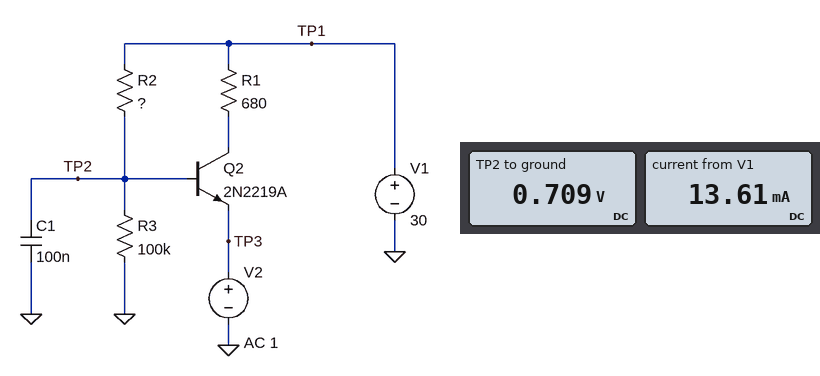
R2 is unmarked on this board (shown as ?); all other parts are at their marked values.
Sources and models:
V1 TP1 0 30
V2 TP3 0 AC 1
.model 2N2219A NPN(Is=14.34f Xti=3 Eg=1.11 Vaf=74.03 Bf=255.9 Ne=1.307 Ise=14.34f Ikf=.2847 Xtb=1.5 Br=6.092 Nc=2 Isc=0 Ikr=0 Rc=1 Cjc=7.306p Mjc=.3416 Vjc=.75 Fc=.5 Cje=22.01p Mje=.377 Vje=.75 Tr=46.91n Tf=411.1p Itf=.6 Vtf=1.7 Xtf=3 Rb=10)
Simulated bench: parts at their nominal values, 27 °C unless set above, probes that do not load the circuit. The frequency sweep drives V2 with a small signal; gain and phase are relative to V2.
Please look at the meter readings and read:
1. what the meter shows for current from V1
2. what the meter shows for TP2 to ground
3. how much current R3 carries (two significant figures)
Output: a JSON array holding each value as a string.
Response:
["13.61 mA", "0.709 V", "7.1 µA"]
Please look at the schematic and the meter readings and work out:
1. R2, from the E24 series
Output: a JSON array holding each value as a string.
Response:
["430 kΩ"]
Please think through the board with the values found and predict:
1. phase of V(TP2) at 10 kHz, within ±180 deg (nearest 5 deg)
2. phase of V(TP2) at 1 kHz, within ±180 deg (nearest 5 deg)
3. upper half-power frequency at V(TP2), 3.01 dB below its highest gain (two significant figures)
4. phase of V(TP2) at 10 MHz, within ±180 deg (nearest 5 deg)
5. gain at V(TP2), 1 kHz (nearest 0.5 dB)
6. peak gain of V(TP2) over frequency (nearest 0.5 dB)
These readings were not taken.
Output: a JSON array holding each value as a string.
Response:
["-70 deg", "-15 deg", "3.4 kHz", "-35 deg", "-0.5 dB", "0 dB"]
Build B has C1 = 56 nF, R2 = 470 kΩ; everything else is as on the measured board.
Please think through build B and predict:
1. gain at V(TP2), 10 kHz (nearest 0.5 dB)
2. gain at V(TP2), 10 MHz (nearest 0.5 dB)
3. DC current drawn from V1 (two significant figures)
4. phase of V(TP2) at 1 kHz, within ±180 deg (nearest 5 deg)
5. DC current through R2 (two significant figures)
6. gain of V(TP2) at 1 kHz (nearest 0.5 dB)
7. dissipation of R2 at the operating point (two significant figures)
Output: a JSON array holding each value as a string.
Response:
["-6.5 dB", "-37.5 dB", "12 mA", "-10 deg", "62 µA", "0 dB", "1.8 mW"]
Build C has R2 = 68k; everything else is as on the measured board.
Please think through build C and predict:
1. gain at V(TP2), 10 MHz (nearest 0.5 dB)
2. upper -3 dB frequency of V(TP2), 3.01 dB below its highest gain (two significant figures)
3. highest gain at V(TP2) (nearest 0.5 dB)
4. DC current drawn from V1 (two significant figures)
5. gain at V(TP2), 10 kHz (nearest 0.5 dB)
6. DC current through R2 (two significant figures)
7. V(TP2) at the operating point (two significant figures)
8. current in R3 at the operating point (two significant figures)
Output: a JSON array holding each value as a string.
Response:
["-36.5 dB", "110 kHz", "0 dB", "44 mA", "0 dB", "430 µA", "750 mV", "7.5 µA"]
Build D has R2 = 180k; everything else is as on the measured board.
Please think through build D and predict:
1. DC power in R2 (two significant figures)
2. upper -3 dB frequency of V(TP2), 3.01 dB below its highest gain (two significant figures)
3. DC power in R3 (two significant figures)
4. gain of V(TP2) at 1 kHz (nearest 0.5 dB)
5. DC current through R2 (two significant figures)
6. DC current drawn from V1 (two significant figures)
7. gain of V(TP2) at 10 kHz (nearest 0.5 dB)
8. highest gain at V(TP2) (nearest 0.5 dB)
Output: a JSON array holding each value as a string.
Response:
["4.8 mW", "8.4 kHz", "5.4 µW", "0 dB", "160 µA", "31 mA", "-4.0 dB", "0 dB"]
